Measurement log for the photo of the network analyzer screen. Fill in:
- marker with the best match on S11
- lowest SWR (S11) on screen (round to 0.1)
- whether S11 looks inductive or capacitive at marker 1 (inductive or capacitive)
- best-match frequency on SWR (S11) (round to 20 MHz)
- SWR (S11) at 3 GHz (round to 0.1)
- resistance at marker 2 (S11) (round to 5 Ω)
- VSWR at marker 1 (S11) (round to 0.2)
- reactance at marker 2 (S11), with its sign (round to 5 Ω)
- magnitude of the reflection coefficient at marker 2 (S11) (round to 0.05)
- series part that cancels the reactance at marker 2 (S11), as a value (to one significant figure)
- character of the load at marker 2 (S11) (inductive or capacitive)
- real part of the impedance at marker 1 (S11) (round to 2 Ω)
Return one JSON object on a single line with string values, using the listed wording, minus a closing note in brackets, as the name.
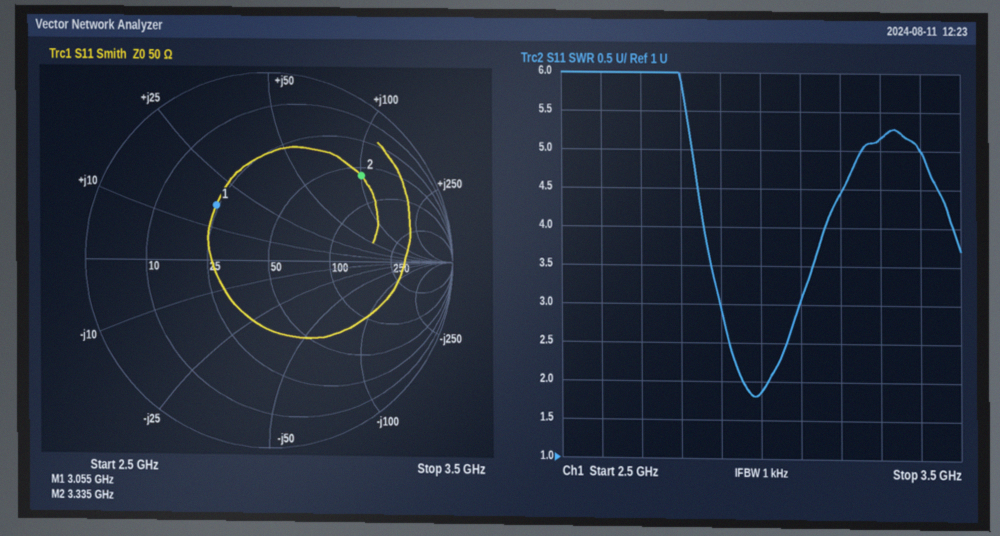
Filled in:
{"marker with the best match on S11": "marker 1", "lowest SWR (S11) on screen": "1.8", "whether S11 looks inductive or capacitive at marker 1": "inductive", "best-match frequency on SWR (S11)": "2.98 GHz", "SWR (S11) at 3 GHz": "1.9", "resistance at marker 2 (S11)": "60 Ω", "VSWR at marker 1 (S11)": "2.4", "reactance at marker 2 (S11), with its sign": "+100 Ω", "magnitude of the reflection coefficient at marker 2 (S11)": "0.70", "series part that cancels the reactance at marker 2 (S11), as a value": "500 fF", "character of the load at marker 2 (S11)": "inductive", "real part of the impedance at marker 1 (S11)": "24 Ω"}
